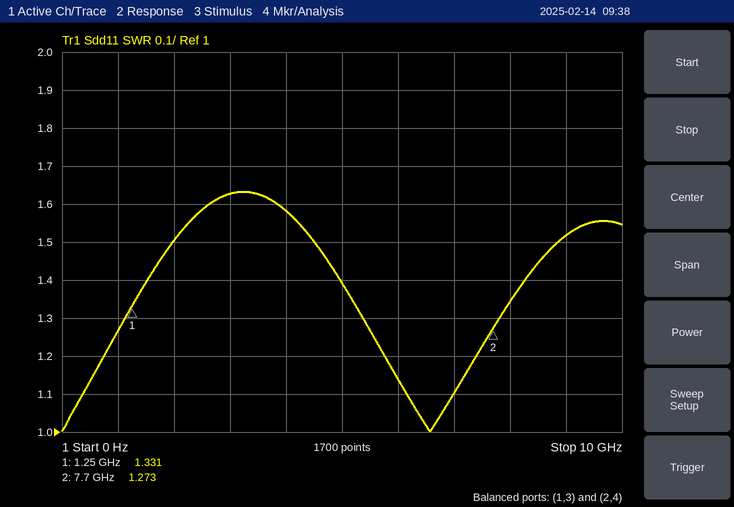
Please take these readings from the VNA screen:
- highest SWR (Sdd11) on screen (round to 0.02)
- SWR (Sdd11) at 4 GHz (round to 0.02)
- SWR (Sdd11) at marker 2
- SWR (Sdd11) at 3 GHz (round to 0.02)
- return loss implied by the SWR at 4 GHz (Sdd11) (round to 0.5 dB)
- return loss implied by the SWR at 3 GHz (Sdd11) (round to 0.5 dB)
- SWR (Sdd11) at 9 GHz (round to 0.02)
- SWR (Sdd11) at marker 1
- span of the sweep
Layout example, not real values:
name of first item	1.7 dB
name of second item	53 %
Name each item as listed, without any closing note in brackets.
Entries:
highest SWR (Sdd11) on screen	1.64
SWR (Sdd11) at 4 GHz	1.58
SWR (Sdd11) at marker 2	1.273
SWR (Sdd11) at 3 GHz	1.62
return loss implied by the SWR at 4 GHz (Sdd11)	13.0 dB
return loss implied by the SWR at 3 GHz (Sdd11)	12.5 dB
SWR (Sdd11) at 9 GHz	1.52
SWR (Sdd11) at marker 1	1.331
span of the sweep	10 GHz
